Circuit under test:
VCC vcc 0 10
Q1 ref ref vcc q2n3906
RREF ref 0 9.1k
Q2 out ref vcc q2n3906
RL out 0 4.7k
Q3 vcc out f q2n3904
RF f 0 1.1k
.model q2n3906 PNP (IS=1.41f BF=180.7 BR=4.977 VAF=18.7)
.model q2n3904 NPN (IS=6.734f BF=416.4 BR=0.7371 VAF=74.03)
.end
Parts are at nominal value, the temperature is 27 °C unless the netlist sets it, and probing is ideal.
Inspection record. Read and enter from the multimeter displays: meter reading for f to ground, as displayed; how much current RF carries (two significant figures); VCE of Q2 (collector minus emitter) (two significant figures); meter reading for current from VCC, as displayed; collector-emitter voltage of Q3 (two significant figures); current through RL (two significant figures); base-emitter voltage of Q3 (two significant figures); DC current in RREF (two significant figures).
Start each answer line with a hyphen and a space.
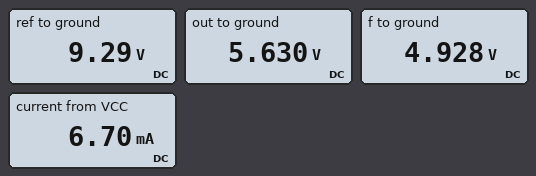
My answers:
- 4.928 V
- 4.5 mA
- -4.4 V
- 6.70 mA
- 5.1 V
- 1.2 mA
- 700 mV
- 1.0 mA
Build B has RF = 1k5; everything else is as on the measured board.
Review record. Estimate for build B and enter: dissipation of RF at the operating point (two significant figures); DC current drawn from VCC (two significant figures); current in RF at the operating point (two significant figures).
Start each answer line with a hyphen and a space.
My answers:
- 16 mW
- 5.5 mA
- 3.3 mA
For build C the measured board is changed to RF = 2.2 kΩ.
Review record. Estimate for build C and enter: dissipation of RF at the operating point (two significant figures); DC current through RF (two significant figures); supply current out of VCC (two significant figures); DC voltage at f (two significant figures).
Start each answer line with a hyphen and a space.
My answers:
- 11 mW
- 2.3 mA
- 4.5 mA
- 5.0 V
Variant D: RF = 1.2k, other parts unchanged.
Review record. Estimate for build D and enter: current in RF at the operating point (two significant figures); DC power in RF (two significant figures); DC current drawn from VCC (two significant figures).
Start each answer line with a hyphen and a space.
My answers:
- 4.1 mA
- 20 mW
- 6.3 mA
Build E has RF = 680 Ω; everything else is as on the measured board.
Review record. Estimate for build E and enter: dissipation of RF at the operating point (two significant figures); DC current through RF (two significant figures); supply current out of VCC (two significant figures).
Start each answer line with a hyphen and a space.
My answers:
- 35 mW
- 7.2 mA
- 9.4 mA
